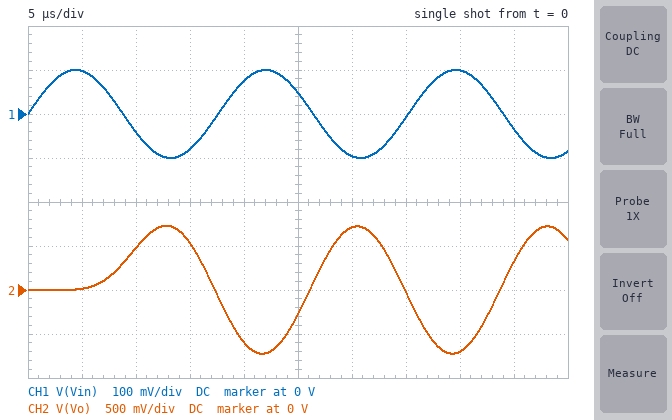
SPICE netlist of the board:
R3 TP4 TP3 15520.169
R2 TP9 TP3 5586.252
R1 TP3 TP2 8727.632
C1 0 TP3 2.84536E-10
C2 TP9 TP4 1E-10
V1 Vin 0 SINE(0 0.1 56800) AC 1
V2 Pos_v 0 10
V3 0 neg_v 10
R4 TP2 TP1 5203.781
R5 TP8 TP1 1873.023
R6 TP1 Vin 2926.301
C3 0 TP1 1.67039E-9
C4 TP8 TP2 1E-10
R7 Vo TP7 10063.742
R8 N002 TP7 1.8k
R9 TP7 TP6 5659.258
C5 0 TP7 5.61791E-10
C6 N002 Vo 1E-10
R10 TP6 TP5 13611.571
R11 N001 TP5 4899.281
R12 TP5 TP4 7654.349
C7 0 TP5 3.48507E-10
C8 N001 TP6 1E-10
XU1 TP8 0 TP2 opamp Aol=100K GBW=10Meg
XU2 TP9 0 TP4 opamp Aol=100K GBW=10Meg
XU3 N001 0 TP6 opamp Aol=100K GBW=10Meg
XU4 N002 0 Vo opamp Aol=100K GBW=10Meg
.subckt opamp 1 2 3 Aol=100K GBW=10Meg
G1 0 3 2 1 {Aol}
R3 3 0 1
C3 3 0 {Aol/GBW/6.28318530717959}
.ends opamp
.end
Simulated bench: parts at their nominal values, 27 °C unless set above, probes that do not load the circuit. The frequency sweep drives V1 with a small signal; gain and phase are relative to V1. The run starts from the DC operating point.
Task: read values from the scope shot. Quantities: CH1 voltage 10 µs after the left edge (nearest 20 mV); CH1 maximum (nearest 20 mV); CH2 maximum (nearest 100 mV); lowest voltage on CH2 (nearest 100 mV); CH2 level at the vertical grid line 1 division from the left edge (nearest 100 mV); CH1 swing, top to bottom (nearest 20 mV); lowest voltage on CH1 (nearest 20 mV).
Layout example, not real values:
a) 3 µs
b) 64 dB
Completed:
a) -40 mV
b) 100 mV
c) 700 mV
d) -700 mV
e) 0 V
f) 200 mV
g) -100 mV
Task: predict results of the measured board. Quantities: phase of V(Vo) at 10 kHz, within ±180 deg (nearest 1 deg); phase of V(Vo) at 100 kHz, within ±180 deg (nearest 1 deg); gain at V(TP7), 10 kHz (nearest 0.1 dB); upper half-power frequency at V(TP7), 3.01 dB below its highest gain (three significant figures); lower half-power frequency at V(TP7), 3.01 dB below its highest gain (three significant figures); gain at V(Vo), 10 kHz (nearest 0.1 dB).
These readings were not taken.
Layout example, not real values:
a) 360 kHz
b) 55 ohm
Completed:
a) -31 deg
b) 54 deg
c) -18.3 dB
d) 110 kHz
e) 34.3 kHz
f) 19.9 dB
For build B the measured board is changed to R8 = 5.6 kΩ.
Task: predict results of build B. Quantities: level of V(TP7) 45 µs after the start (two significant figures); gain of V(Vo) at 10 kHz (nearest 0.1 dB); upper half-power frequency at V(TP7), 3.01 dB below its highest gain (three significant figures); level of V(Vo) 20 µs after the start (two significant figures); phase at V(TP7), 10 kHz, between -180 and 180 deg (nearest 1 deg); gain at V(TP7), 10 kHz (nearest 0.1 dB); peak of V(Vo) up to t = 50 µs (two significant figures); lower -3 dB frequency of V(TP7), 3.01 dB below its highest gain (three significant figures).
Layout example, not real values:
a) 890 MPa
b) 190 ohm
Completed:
a) -140 mV
b) 19.9 dB
c) 94.4 kHz
d) -340 mV
e) -125 deg
f) -8.9 dB
g) 680 mV
h) 29.9 kHz
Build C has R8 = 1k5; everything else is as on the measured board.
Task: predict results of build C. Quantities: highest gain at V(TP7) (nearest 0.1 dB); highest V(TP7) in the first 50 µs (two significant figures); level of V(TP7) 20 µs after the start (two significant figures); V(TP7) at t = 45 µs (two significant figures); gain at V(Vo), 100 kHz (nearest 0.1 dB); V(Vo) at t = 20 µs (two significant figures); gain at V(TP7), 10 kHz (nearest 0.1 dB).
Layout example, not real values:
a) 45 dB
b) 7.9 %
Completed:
a) -7.0 dB
b) 43 mV
c) 23 mV
d) -37 mV
e) 11.1 dB
f) -610 mV
g) -19.7 dB
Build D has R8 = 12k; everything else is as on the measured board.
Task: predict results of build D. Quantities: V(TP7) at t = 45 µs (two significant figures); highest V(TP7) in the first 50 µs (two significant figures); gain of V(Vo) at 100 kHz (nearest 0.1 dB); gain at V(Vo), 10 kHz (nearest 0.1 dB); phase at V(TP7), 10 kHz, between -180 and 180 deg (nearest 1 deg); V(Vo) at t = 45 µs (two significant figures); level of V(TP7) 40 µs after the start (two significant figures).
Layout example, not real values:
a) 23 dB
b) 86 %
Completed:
a) -180 mV
b) 210 mV
c) 1.8 dB
d) 19.8 dB
e) -131 deg
f) -210 mV
g) 130 mV
